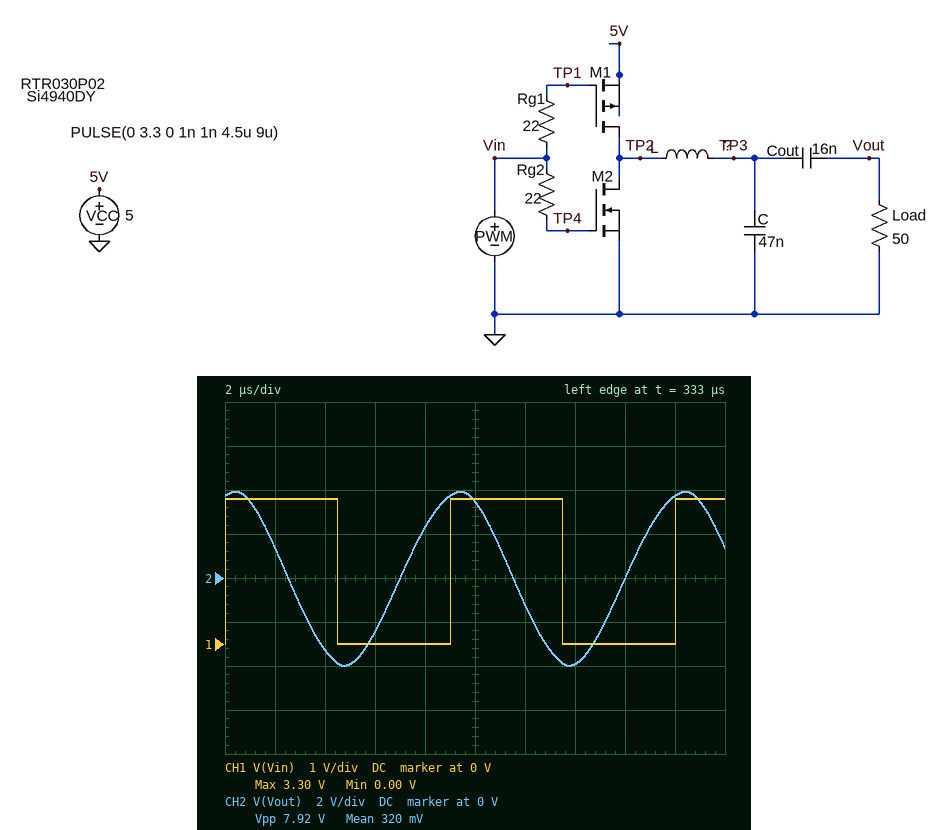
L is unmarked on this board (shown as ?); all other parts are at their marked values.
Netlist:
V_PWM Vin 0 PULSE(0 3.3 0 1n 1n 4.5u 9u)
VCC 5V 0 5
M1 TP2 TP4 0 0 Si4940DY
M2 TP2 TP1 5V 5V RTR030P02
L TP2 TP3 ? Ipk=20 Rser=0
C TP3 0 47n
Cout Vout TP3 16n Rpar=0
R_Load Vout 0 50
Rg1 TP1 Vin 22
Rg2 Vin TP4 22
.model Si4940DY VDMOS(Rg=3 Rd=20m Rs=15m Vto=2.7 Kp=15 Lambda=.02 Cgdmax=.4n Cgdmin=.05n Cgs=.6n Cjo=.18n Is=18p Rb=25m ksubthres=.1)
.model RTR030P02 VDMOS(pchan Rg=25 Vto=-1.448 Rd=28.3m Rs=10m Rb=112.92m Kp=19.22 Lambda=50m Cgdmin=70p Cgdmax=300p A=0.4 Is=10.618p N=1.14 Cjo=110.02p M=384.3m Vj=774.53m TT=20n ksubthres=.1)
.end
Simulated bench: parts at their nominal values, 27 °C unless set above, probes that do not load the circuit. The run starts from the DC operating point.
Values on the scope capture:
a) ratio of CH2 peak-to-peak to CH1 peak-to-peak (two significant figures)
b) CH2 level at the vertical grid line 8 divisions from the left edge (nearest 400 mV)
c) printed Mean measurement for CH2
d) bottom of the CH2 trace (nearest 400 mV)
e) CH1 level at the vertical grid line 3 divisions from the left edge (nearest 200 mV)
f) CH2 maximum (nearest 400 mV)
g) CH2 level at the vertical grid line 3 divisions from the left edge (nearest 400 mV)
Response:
2.4
0 V
320 mV
-4.0 V
0 V
4.0 V
-2.4 V
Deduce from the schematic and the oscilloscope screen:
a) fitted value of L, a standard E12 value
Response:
47 µH
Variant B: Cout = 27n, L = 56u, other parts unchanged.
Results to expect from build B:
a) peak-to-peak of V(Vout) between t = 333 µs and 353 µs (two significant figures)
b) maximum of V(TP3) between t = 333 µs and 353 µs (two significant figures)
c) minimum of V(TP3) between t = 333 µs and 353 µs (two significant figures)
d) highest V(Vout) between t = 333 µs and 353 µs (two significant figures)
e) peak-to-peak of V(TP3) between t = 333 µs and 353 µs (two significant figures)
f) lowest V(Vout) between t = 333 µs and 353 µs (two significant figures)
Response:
5.7 V
6.8 V
-1.2 V
2.8 V
8.0 V
-2.9 V
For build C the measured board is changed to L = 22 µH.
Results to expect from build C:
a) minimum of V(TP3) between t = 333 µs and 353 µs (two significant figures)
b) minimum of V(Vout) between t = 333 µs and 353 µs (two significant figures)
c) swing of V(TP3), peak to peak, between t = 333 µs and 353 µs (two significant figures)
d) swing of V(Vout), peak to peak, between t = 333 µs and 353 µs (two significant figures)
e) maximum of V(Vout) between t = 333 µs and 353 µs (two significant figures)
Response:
-5.4 V
-3.8 V
17 V
8.1 V
4.2 V
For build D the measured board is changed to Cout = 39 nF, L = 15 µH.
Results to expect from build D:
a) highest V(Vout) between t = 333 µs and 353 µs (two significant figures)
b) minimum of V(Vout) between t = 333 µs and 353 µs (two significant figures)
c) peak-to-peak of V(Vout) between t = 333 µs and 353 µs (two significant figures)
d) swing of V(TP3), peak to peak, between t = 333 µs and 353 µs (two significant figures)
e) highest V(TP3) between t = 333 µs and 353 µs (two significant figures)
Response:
5.1 V
-4.2 V
9.3 V
11 V
8.7 V
